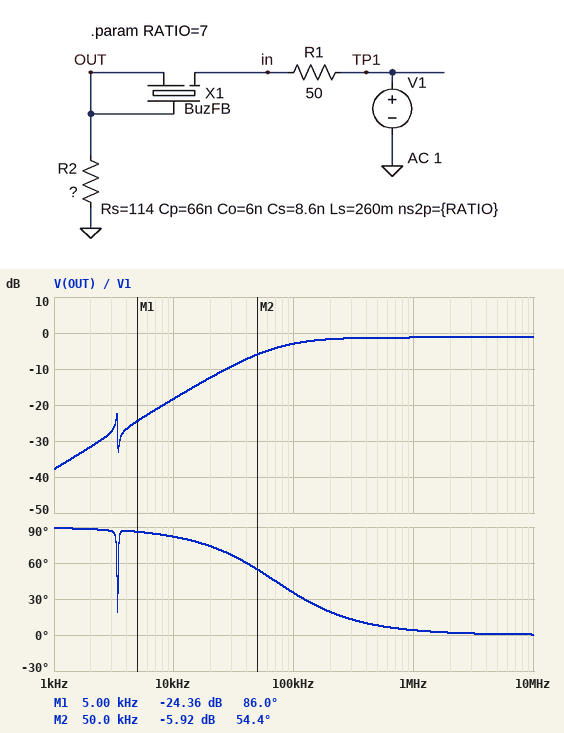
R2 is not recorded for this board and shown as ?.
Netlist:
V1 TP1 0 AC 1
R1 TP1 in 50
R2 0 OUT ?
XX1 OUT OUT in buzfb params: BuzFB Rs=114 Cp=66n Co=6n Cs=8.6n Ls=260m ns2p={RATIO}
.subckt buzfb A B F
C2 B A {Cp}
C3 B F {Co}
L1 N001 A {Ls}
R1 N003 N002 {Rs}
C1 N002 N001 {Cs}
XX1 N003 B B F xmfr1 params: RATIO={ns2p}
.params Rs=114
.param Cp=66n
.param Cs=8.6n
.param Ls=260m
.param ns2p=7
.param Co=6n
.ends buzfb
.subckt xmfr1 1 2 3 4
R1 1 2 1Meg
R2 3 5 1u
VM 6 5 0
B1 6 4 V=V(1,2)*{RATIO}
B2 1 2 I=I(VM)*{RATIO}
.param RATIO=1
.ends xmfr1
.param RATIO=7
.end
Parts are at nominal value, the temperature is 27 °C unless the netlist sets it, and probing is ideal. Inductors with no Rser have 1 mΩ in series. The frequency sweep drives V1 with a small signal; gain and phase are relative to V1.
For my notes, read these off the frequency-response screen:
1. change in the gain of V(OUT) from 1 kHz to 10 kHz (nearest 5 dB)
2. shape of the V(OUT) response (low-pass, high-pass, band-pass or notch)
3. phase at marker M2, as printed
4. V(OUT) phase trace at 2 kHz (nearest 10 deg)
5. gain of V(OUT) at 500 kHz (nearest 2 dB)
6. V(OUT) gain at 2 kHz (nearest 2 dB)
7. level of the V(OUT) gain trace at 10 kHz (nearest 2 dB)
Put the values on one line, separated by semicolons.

20 dB; high-pass; 54.4 deg; 90 deg; -2 dB; -32 dB; -18 dB
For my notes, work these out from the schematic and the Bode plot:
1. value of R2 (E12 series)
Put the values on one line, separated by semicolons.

330 Ω
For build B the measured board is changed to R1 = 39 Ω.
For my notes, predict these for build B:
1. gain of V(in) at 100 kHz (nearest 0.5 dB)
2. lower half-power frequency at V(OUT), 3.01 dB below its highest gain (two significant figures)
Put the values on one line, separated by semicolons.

-0.5 dB; 72 kHz
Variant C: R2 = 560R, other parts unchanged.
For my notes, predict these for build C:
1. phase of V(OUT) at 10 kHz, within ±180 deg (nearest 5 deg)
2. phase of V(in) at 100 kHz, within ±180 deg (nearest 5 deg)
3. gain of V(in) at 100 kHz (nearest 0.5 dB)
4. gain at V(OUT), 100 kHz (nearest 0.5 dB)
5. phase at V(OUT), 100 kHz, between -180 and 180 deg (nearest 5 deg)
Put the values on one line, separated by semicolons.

75 deg; 0 deg; -0.5 dB; -1.5 dB; 25 deg
